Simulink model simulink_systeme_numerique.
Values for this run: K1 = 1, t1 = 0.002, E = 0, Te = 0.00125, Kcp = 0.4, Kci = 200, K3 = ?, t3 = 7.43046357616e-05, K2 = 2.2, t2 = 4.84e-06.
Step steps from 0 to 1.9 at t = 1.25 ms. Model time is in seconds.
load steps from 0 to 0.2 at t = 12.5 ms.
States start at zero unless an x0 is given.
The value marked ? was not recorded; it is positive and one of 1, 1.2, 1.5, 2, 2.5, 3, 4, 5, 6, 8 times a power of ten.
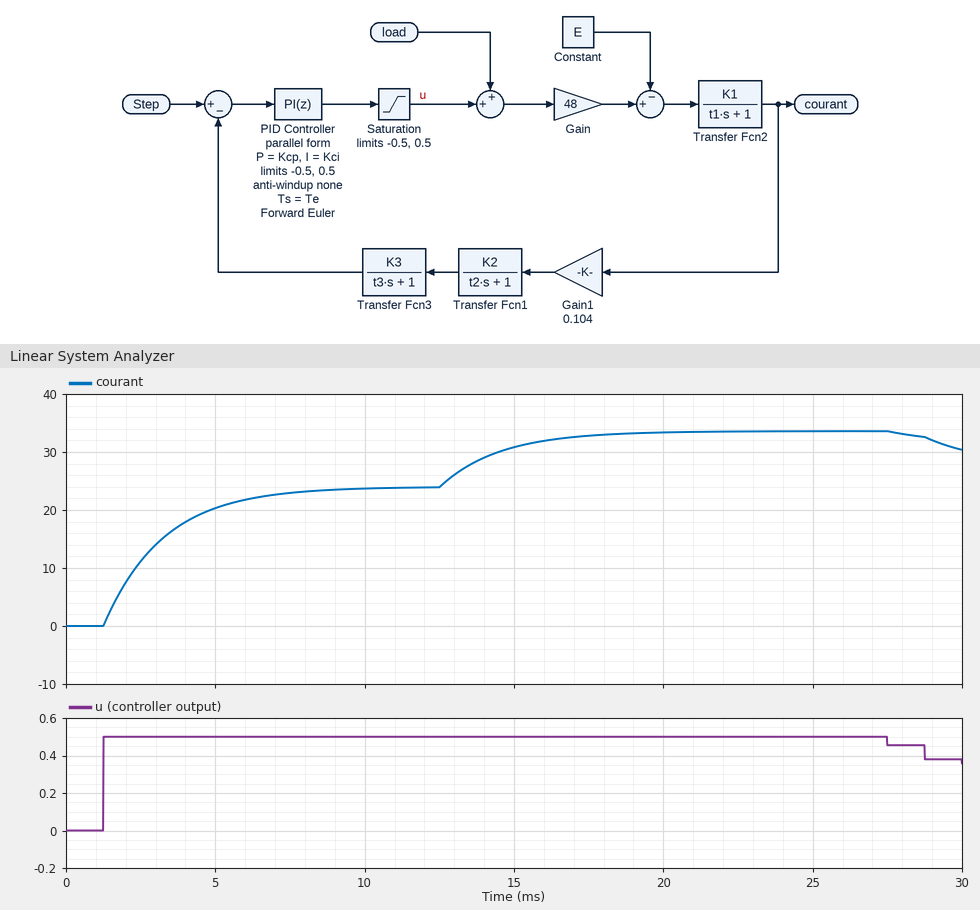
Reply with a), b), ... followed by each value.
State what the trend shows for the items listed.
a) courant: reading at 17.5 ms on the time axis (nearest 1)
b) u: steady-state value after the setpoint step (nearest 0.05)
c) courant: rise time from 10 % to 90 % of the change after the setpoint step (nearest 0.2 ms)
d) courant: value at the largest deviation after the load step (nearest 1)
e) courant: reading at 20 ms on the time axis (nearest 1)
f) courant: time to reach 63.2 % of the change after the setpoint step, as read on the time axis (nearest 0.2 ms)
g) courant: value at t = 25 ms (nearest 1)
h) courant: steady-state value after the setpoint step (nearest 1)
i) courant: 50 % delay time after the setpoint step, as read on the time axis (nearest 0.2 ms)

a) 33
b) 0.50
c) 4.4 ms
d) 34
e) 33
f) 3.2 ms
g) 34
h) 24
i) 2.6 ms
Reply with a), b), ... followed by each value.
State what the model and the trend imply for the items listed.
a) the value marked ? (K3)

a) 0.3
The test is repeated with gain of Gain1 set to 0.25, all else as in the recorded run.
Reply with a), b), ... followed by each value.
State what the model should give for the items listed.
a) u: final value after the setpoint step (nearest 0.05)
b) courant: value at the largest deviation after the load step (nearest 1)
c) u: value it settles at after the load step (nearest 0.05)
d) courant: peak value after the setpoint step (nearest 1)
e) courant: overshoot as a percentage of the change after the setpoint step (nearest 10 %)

a) 0.25
b) 16
c) 0.05
d) 17
e) 50 %
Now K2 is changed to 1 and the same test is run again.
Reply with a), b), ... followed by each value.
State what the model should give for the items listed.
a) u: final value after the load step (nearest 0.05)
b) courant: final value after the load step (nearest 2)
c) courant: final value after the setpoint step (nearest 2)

a) 0.50
b) 34
c) 24
